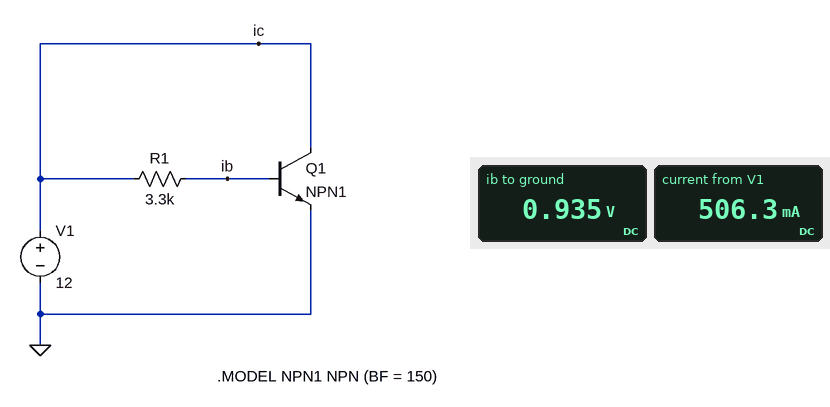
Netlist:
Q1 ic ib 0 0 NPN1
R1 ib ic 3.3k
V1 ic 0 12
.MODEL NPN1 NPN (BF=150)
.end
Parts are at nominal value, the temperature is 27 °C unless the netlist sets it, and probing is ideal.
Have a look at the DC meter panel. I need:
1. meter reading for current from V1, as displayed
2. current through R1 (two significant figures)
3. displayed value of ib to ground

506.3 mA
3.4 mA
0.935 V
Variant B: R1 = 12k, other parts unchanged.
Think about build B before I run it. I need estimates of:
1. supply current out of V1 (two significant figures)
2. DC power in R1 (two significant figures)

140 mA
10 mW
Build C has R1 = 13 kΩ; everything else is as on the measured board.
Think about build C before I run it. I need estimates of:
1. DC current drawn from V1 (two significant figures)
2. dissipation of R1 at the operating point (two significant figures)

130 mA
9.5 mW
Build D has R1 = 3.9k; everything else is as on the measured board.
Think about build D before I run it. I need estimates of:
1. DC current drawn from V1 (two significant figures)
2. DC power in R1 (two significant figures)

430 mA
31 mW
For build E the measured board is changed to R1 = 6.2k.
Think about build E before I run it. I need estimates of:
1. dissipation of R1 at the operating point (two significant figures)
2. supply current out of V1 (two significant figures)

20 mW
270 mA
